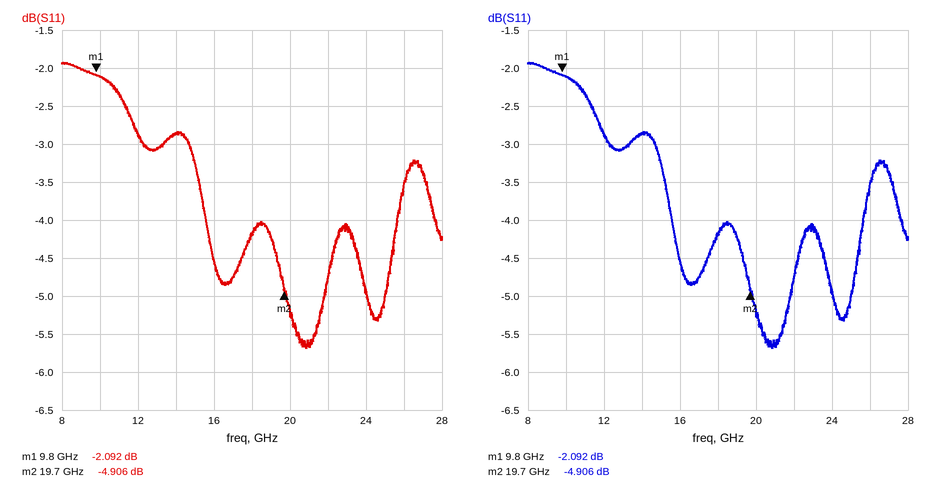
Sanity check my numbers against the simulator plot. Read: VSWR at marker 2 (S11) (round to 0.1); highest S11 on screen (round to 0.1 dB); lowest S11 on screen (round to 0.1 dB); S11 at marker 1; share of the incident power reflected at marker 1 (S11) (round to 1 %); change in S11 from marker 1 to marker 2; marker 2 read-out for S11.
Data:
3.6
-1.9 dB
-5.7 dB
-2.092 dB
62 %
-2.814 dB
-4.906 dB
